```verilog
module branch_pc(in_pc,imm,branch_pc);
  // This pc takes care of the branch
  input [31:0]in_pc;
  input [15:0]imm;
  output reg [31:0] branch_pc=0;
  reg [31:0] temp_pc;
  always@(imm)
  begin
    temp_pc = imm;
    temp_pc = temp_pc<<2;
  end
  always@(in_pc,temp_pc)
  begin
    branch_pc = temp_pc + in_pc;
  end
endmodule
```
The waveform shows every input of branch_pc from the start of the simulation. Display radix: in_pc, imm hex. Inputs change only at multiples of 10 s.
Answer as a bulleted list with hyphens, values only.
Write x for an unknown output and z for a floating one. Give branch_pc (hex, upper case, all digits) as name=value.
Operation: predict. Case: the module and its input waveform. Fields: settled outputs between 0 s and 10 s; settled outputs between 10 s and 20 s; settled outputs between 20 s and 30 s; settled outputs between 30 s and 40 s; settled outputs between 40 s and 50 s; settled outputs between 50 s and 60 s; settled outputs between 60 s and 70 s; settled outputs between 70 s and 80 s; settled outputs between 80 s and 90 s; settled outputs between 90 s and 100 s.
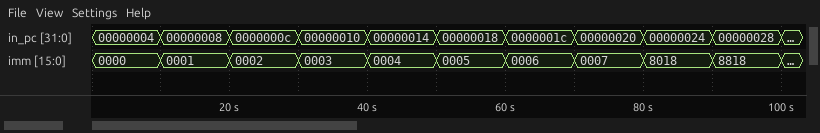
- branch_pc=00000004
- branch_pc=0000000C
- branch_pc=00000014
- branch_pc=0000001C
- branch_pc=00000024
- branch_pc=0000002C
- branch_pc=00000034
- branch_pc=0000003C
- branch_pc=00020084
- branch_pc=00022088
